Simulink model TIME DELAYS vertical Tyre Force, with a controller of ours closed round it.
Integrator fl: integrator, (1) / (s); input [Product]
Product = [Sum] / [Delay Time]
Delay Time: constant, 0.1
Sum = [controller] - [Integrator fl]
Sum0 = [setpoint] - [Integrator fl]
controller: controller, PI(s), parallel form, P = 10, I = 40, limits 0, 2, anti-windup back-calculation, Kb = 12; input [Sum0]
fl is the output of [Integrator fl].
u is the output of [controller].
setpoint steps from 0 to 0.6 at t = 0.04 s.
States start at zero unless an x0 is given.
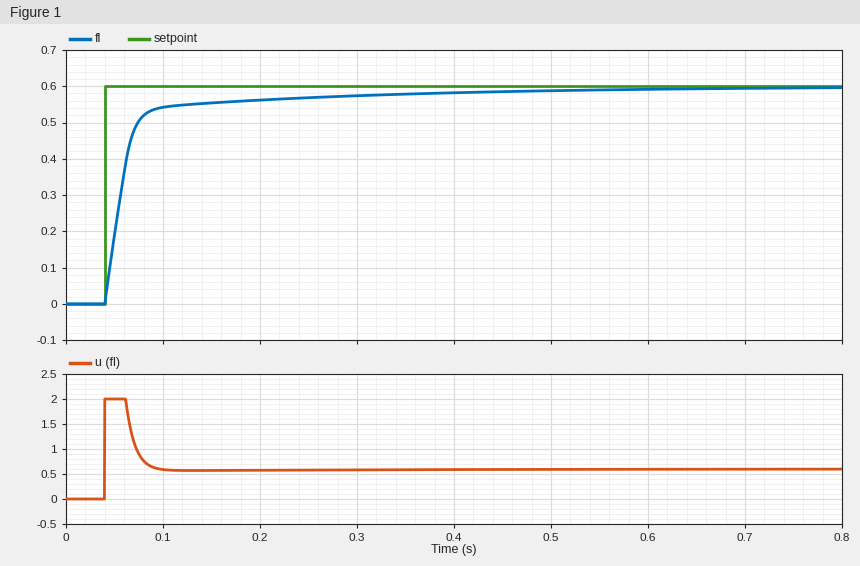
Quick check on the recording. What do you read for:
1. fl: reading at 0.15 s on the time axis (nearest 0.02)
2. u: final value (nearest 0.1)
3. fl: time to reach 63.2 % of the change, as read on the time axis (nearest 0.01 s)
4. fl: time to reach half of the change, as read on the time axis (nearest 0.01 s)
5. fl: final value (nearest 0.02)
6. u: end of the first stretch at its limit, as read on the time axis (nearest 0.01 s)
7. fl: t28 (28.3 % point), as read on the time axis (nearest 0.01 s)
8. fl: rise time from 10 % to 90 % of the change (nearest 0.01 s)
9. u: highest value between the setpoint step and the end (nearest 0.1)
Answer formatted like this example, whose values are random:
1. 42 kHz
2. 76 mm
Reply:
1. 0.56
2. 0.6
3. 0.06 s
4. 0.06 s
5. 0.60
6. 0.06 s
7. 0.05 s
8. 0.05 s
9. 2.0
